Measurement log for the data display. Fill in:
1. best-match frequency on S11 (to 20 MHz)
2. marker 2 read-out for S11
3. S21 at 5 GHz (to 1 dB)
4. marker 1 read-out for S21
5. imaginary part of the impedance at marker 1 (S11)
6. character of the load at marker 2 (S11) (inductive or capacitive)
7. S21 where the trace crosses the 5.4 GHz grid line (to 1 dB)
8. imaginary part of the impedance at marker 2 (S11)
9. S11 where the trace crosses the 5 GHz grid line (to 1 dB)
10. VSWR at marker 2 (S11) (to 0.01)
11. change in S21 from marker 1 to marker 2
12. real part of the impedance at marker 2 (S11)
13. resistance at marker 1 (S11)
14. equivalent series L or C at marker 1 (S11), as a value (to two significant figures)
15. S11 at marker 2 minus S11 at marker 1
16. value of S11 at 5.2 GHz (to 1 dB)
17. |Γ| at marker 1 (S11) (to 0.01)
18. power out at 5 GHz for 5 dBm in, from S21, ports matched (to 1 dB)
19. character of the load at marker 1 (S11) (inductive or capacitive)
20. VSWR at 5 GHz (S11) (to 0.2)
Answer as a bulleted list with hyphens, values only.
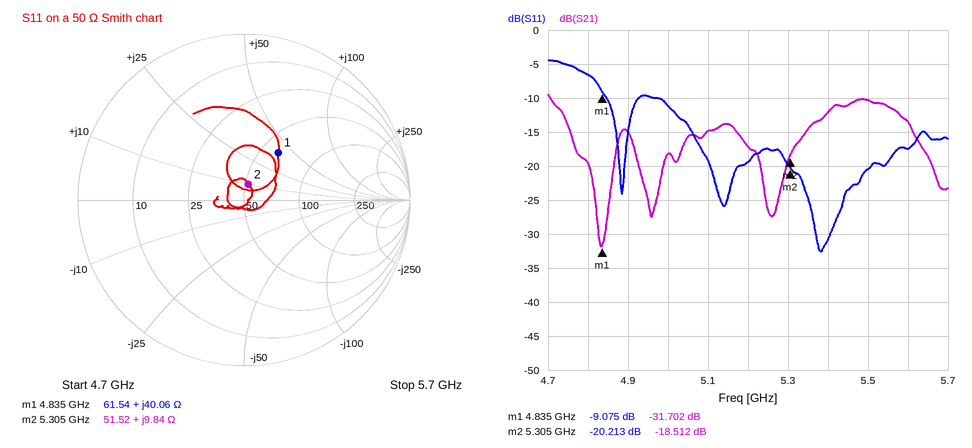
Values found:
- 5.38 GHz
- -20.213 dB
- -18 dB
- -31.702 dB
- +40.06 Ω
- inductive
- -12 dB
- +9.84 Ω
- -11 dB
- 1.22
- 13.190 dB
- 51.52 Ω
- 61.54 Ω
- 1.3 nH
- -11.138 dB
- -19 dB
- 0.35
- -13 dBm
- inductive
- 1.8
